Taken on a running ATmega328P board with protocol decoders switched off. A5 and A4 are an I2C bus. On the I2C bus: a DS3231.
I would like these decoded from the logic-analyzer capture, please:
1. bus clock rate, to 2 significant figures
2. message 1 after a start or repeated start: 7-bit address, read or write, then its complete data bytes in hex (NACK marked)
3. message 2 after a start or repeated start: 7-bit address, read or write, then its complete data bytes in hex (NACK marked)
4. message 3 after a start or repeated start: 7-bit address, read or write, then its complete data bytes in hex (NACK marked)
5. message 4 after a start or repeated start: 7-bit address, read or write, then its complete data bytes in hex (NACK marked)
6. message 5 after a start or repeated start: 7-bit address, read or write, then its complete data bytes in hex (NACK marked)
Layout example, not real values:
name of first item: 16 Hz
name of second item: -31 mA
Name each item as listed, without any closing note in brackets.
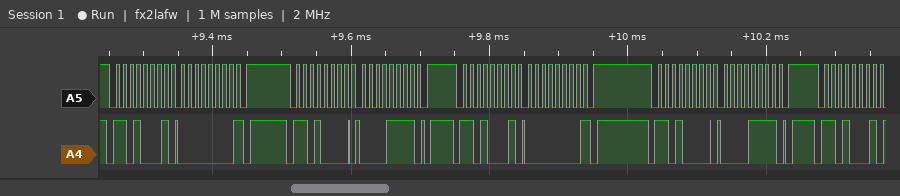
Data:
bus clock rate, to 2 significant figures: 100 kHz
message 1 after a start or repeated start: 7-bit address, read or write, then its complete data bytes in hex: 0x68 read: 00 NACK
message 2 after a start or repeated start: 7-bit address, read or write, then its complete data bytes in hex: 0x68 write: 0F
message 3 after a start or repeated start: 7-bit address, read or write, then its complete data bytes in hex: 0x68 read: 00 NACK
message 4 after a start or repeated start: 7-bit address, read or write, then its complete data bytes in hex: 0x68 write: 0F
message 5 after a start or repeated start: 7-bit address, read or write, then its complete data bytes in hex: 0x68 read
